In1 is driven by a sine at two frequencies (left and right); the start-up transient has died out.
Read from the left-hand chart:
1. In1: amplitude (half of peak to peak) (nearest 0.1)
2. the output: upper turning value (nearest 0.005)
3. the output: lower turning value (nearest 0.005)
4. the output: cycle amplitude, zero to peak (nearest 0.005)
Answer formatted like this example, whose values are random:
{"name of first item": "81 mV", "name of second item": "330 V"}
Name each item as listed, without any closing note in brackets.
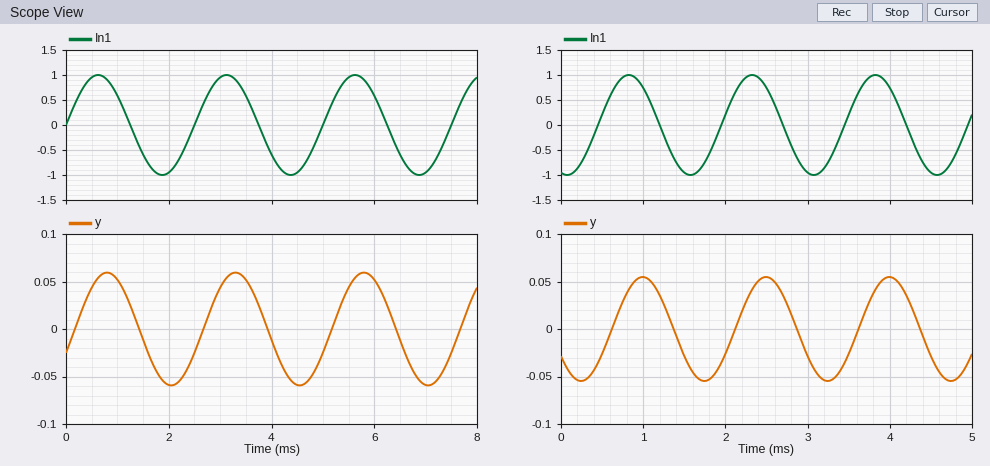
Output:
{"In1: amplitude (half of peak to peak)": "1.0", "the output: upper turning value": "0.060", "the output: lower turning value": "-0.060", "the output: cycle amplitude, zero to peak": "0.060"}
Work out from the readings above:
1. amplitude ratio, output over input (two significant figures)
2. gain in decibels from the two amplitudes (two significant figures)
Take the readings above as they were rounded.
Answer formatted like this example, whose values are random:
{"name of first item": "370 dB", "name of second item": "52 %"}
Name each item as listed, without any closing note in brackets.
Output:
{"amplitude ratio, output over input": "0.060", "gain in decibels from the two amplitudes": "-24 dB"}
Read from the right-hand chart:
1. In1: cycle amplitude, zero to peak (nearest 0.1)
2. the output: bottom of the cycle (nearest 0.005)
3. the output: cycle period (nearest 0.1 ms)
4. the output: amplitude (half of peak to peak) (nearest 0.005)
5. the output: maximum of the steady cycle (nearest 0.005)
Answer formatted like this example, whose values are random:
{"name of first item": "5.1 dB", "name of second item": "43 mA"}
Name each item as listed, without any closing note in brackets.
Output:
{"In1: cycle amplitude, zero to peak": "1.0", "the output: bottom of the cycle": "-0.055", "the output: cycle period": "1.5 ms", "the output: amplitude (half of peak to peak)": "0.055", "the output: maximum of the steady cycle": "0.055"}
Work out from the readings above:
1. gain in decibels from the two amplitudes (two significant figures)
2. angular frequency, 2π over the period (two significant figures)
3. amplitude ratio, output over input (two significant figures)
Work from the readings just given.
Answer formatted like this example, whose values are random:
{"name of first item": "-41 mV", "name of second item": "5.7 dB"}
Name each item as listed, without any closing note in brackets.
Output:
{"gain in decibels from the two amplitudes": "-25 dB", "angular frequency, 2π over the period": "4.2 rad/ms", "amplitude ratio, output over input": "0.055"}
